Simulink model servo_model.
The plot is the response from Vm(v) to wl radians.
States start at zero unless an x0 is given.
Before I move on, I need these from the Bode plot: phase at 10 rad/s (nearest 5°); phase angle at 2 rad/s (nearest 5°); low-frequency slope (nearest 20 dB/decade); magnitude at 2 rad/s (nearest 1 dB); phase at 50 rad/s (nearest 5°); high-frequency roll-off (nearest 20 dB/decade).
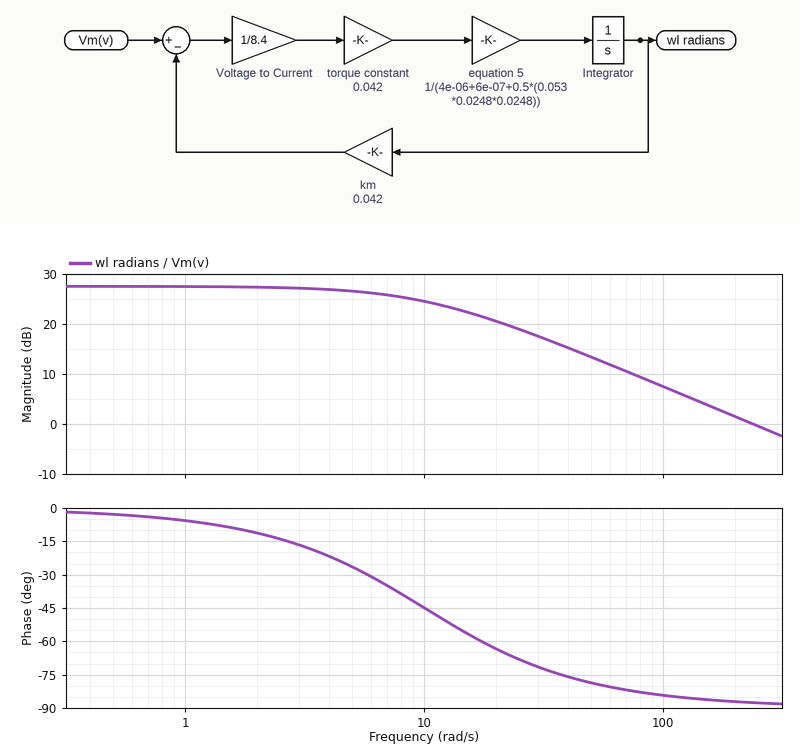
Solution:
-45°
-10°
0 dB/decade
27 dB
-80°
-20 dB/decade
